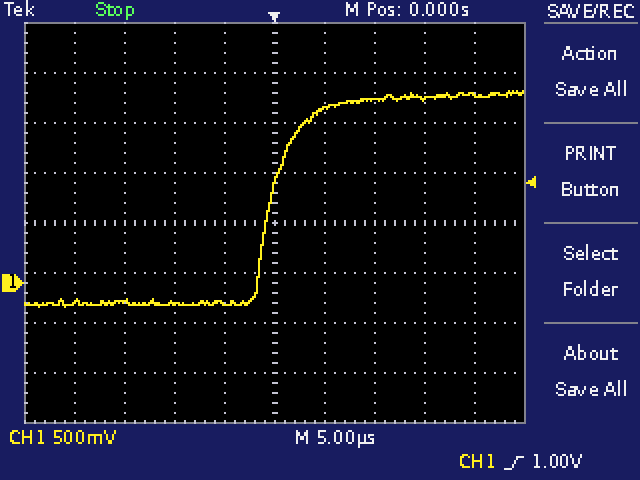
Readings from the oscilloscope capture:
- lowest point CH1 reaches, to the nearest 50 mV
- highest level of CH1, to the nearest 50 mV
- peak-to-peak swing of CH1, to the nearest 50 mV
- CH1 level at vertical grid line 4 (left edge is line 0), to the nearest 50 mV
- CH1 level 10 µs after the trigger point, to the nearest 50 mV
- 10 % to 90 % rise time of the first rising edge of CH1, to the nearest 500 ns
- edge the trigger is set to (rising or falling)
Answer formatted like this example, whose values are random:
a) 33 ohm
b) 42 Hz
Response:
a) -250 mV
b) 1.90 V
c) 2.15 V
d) -200 mV
e) 1.85 V
f) 5.5 µs
g) rising
